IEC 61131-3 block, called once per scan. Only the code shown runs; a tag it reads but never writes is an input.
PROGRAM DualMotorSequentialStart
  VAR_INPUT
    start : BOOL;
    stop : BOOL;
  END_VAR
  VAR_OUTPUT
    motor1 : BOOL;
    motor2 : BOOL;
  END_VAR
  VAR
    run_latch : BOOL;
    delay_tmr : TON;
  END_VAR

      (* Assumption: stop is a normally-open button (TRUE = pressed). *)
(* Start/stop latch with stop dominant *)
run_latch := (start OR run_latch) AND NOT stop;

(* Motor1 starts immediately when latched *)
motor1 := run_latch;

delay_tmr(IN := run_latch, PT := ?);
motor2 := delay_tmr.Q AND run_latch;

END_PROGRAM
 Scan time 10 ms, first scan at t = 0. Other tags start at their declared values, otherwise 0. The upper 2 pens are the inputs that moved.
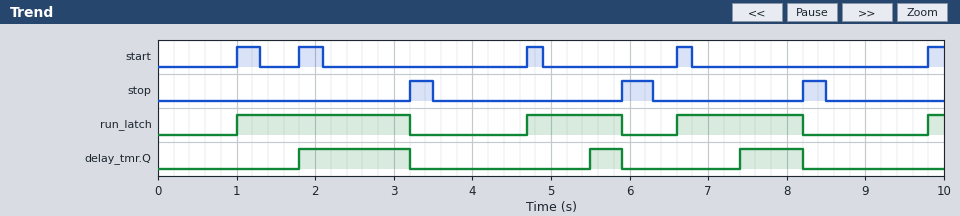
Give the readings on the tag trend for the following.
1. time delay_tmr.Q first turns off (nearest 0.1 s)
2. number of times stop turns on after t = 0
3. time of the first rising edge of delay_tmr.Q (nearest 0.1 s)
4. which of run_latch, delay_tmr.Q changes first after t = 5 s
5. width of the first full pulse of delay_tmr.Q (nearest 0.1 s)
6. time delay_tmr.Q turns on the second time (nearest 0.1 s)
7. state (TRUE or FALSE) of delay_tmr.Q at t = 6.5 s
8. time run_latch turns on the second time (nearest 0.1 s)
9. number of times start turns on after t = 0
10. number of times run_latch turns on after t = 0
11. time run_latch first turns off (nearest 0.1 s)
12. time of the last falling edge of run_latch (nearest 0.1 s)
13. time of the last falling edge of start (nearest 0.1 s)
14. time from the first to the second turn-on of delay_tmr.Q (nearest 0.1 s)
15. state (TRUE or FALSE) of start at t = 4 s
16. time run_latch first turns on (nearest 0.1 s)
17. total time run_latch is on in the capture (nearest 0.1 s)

3.2 s
3
1.8 s
delay_tmr.Q
1.4 s
5.5 s
FALSE
4.7 s
5
4
3.2 s
8.2 s
6.8 s
3.7 s
FALSE
1.0 s
5.2 s
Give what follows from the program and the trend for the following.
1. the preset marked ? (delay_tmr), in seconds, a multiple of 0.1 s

0.8 s
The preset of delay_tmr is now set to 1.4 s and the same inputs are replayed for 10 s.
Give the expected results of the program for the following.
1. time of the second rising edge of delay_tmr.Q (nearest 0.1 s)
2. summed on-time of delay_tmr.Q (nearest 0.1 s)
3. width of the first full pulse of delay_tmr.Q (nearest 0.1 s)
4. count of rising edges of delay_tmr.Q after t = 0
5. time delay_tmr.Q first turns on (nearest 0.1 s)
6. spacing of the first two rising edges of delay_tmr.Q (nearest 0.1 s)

8.0 s
1.0 s
0.8 s
2
2.4 s
5.6 s
